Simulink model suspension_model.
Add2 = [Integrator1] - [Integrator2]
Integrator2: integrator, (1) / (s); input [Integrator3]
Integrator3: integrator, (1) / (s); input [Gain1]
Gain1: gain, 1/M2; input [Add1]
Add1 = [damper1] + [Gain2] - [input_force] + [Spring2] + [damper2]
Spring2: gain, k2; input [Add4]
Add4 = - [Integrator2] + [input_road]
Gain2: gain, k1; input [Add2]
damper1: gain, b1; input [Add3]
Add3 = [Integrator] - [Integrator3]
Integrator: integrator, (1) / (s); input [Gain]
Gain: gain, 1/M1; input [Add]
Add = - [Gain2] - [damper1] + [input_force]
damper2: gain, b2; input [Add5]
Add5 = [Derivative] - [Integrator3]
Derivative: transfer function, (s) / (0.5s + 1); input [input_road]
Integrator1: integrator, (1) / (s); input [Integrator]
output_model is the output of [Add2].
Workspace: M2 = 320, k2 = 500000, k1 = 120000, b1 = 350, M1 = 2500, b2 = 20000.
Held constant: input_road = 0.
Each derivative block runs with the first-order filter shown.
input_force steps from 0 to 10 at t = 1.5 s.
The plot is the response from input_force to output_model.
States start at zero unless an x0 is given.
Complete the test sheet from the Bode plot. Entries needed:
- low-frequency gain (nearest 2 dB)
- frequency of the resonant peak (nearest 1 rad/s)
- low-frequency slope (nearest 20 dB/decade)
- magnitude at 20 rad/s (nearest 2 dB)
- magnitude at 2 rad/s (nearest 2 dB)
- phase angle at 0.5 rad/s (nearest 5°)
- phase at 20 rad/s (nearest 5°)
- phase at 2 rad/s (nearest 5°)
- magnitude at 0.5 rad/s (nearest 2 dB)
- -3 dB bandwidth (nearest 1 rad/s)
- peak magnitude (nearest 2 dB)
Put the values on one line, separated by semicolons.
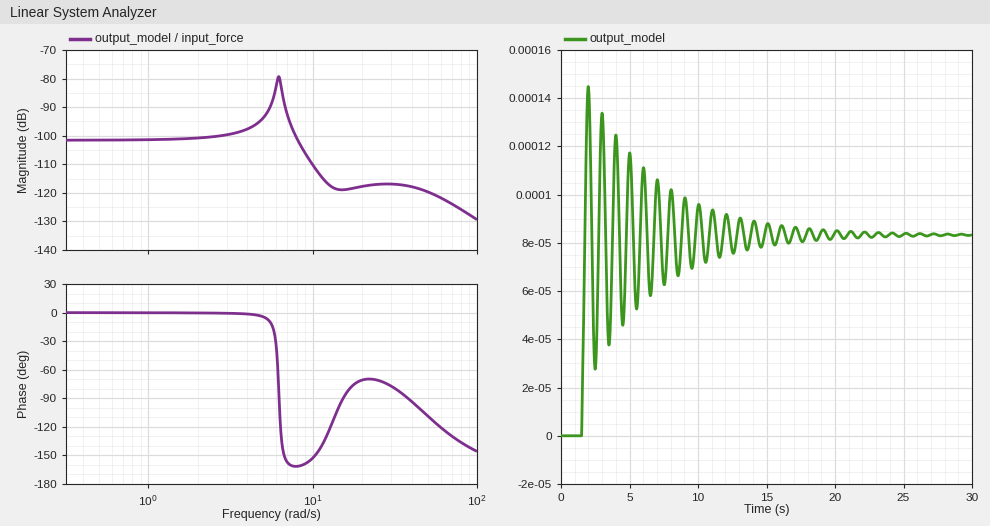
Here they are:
-102 dB; 6 rad/s; 0 dB/decade; -118 dB; -100 dB; 0°; -70°; 0°; -102 dB; 9 rad/s; -80 dB
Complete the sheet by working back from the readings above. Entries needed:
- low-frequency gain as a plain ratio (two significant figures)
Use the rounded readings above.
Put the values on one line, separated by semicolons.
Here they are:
0.0000079
